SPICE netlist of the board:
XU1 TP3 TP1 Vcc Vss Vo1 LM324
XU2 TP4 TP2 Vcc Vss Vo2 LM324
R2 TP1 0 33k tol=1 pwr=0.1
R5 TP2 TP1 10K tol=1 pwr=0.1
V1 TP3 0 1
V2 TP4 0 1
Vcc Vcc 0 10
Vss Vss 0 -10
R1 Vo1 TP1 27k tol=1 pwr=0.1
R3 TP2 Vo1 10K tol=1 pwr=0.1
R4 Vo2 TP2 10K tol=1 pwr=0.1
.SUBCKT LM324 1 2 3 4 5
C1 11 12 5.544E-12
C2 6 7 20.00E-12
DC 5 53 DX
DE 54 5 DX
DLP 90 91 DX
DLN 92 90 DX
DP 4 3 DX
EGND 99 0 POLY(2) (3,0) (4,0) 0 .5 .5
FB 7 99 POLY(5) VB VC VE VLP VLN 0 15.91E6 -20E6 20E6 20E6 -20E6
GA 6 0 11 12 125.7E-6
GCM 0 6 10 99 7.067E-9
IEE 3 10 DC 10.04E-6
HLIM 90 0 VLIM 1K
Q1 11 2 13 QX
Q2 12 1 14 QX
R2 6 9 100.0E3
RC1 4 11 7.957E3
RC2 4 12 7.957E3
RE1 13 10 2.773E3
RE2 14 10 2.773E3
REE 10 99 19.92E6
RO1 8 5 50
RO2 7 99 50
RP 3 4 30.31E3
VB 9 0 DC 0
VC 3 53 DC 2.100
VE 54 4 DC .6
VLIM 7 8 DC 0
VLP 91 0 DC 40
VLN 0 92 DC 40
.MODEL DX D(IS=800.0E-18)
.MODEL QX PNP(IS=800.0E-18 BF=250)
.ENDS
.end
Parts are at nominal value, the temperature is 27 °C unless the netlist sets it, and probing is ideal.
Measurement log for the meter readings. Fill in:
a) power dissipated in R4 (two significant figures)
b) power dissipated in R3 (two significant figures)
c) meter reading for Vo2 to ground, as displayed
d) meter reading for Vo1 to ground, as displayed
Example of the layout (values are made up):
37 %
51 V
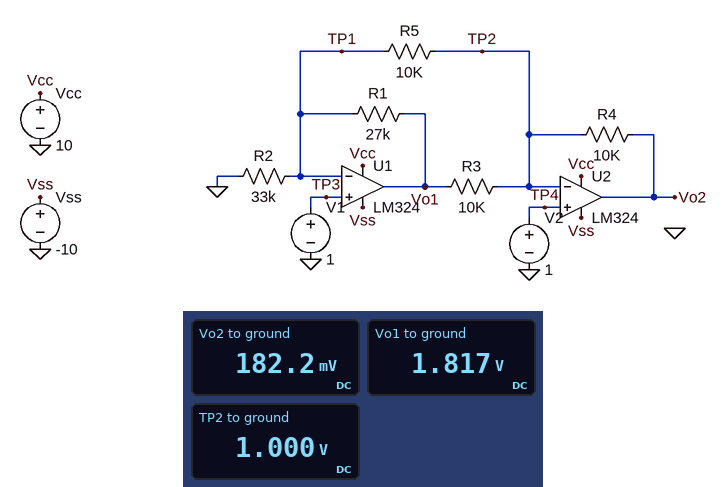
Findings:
67 µW
67 µW
182.2 mV
1.817 V
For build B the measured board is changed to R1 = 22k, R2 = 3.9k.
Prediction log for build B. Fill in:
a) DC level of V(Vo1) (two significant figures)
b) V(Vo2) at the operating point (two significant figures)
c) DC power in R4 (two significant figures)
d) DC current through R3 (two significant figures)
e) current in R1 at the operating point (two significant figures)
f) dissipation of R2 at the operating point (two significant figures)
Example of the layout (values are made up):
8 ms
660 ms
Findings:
6.6 V
-4.6 V
3.2 mW
560 µA
260 µA
260 µW
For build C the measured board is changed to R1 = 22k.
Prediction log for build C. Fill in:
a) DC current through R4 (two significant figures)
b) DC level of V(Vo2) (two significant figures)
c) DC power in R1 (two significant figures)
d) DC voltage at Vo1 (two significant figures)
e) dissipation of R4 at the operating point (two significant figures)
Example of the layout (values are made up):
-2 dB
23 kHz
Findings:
67 µA
330 mV
20 µW
1.7 V
44 µW
